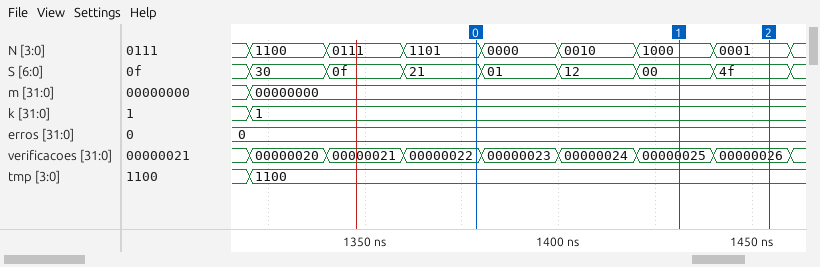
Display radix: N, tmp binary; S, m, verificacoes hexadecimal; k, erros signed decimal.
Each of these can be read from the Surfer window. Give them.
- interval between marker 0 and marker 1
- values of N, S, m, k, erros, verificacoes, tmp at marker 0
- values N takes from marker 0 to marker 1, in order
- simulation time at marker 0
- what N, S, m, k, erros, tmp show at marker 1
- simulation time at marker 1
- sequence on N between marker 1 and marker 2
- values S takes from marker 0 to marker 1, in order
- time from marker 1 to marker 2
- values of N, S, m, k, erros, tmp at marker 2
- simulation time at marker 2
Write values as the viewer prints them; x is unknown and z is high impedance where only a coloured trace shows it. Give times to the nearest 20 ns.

60 ns
N=1101, S=21, m=00000000, k=1, erros=0, verificacoes=00000022, tmp=1100
1101, 0000, 0010, 1000
1380 ns
N=1000, S=00, m=00000000, k=1, erros=0, tmp=1100
1440 ns
1000, 0001
21, 01, 12, 00
20 ns
N=0001, S=4f, m=00000000, k=1, erros=0, tmp=1100
1460 ns
